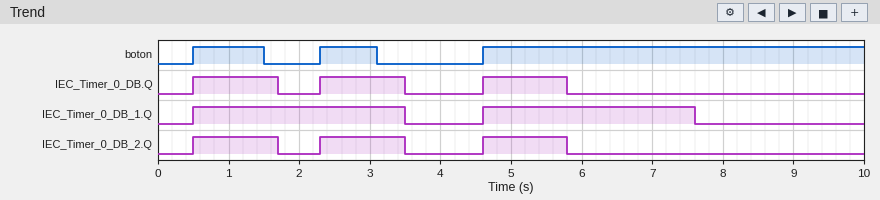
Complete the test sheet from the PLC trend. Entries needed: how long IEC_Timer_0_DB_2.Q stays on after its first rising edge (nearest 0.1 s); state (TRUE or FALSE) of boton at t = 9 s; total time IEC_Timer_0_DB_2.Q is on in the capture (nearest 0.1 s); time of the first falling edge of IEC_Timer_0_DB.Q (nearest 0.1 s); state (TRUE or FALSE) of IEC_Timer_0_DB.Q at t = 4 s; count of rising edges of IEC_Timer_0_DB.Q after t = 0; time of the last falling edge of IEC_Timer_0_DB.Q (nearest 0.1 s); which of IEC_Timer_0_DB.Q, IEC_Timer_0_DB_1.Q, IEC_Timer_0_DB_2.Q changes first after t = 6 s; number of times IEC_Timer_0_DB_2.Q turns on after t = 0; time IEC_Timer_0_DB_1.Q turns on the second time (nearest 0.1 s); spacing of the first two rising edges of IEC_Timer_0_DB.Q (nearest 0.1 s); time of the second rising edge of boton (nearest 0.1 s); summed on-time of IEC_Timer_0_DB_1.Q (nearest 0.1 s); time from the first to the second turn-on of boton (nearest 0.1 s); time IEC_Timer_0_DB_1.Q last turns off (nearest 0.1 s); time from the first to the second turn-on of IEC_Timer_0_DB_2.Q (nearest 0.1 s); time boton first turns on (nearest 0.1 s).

1.2 s
TRUE
3.6 s
1.7 s
FALSE
3
5.8 s
IEC_Timer_0_DB_1.Q
3
4.6 s
1.8 s
2.3 s
6.0 s
1.8 s
7.6 s
1.8 s
0.5 s
